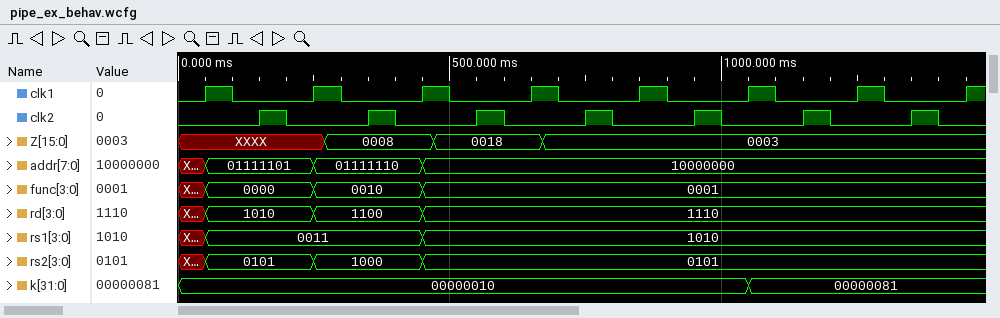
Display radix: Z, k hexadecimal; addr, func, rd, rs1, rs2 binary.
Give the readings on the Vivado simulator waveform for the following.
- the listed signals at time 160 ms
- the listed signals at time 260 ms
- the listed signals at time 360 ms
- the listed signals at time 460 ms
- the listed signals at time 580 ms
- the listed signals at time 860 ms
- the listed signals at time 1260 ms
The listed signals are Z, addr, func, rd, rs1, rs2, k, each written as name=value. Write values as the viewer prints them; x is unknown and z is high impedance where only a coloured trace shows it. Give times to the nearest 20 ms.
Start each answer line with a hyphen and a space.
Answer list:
- Z=XXXX, addr=01111101, func=0000, rd=1010, rs1=0011, rs2=0101, k=00000010
- Z=XXXX, addr=01111110, func=0010, rd=1100, rs1=0011, rs2=1000, k=00000010
- Z=0008, addr=01111110, func=0010, rd=1100, rs1=0011, rs2=1000, k=00000010
- Z=0008, addr=10000000, func=0001, rd=1110, rs1=1010, rs2=0101, k=00000010
- Z=0018, addr=10000000, func=0001, rd=1110, rs1=1010, rs2=0101, k=00000010
- Z=0003, addr=10000000, func=0001, rd=1110, rs1=1010, rs2=0101, k=00000010
- Z=0003, addr=10000000, func=0001, rd=1110, rs1=1010, rs2=0101, k=00000081
